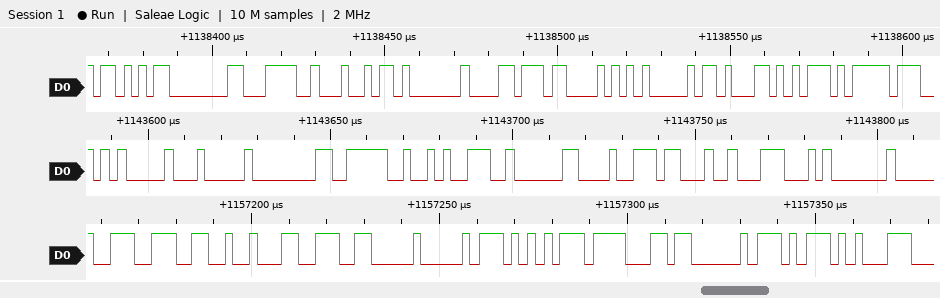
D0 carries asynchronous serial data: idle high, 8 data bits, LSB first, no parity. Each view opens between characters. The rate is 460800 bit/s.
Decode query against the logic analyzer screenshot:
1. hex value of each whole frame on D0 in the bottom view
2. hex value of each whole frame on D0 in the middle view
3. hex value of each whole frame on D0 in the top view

CE, 26, CC, 06, D0, D5, 8F, 03, D7, C5
05, 04, 80, 3E, CA, 02, C8, 23, 1C, 01
AB, 80, 3C, A4, 01, D8, 43, 05, 8B, 75, DF
